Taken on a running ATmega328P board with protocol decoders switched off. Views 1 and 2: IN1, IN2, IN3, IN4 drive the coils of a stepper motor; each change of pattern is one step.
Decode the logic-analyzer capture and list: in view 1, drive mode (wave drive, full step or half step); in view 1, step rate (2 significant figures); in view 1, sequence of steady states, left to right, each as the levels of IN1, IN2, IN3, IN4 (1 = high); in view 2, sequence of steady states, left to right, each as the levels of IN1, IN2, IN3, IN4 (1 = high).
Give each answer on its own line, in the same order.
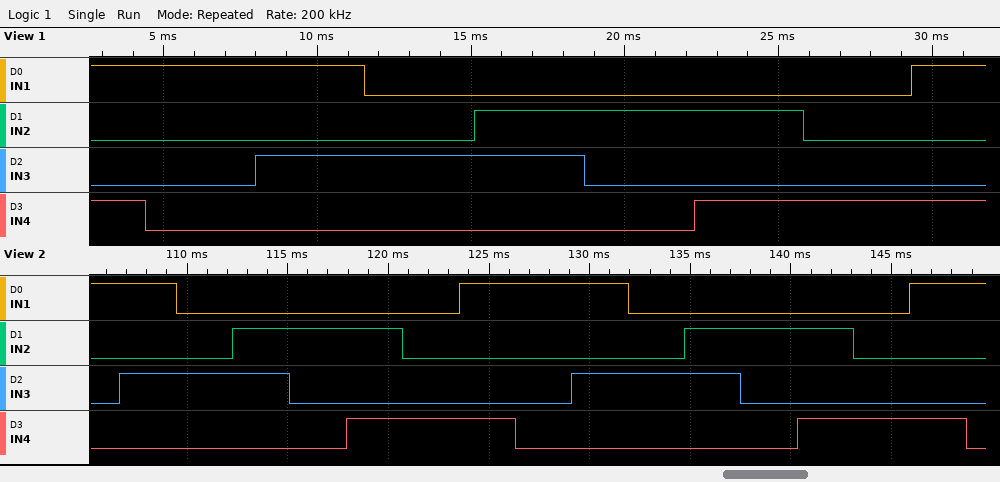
half step
280 steps/s
1001 1000 1010 0010 0110 0100 0101 0001 1001
1000 1010 0010 0110 0100 0101 0001 1001 1000 1010 0010 0110 0100 0101 0001 1001 1000
